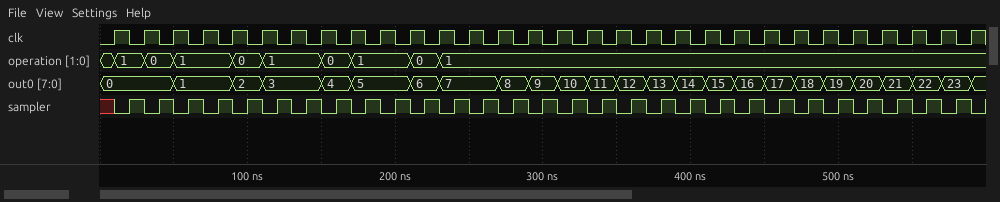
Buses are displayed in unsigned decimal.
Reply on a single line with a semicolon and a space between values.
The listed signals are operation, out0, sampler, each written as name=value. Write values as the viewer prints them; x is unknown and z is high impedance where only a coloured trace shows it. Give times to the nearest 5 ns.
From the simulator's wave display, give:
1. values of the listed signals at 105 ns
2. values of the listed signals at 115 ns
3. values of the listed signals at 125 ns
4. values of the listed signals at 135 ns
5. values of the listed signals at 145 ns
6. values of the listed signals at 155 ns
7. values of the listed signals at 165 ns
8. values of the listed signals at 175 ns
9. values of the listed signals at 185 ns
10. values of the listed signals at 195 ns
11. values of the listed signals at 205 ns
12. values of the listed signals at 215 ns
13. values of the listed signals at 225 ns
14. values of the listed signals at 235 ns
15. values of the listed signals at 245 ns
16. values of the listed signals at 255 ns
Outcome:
operation=0, out0=2, sampler=1; operation=1, out0=3, sampler=0; operation=1, out0=3, sampler=1; operation=1, out0=3, sampler=0; operation=1, out0=3, sampler=1; operation=0, out0=4, sampler=0; operation=0, out0=4, sampler=1; operation=1, out0=5, sampler=0; operation=1, out0=5, sampler=1; operation=1, out0=5, sampler=0; operation=1, out0=5, sampler=1; operation=0, out0=6, sampler=0; operation=0, out0=6, sampler=1; operation=1, out0=7, sampler=0; operation=1, out0=7, sampler=1; operation=1, out0=7, sampler=0
